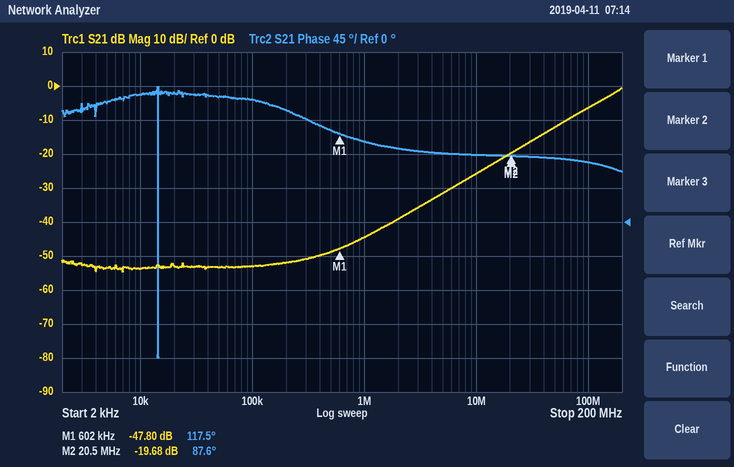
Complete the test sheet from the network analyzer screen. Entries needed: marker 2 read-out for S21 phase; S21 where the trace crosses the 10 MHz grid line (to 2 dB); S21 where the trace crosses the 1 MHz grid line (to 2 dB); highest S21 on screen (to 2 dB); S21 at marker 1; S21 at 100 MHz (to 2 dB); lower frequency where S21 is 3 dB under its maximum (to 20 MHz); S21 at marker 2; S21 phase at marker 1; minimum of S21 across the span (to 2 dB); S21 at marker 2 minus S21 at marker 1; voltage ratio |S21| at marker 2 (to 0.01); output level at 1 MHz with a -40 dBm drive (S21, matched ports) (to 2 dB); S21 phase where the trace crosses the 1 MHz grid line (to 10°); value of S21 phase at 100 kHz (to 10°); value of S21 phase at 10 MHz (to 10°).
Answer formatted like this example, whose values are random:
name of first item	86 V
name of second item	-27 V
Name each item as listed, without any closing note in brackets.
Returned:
marker 2 read-out for S21 phase	87.6°
S21 where the trace crosses the 10 MHz grid line	-26 dB
S21 where the trace crosses the 1 MHz grid line	-44 dB
highest S21 on screen	0 dB
S21 at marker 1	-47.80 dB
S21 at 100 MHz	-6 dB
lower frequency where S21 is 3 dB under its maximum	140 MHz
S21 at marker 2	-19.68 dB
S21 phase at marker 1	117.5°
minimum of S21 across the span	-54 dB
S21 at marker 2 minus S21 at marker 1	28.12 dB
voltage ratio |S21| at marker 2	0.10
output level at 1 MHz with a -40 dBm drive (S21, matched ports)	-84 dBm
S21 phase where the trace crosses the 1 MHz grid line	110°
value of S21 phase at 100 kHz	160°
value of S21 phase at 10 MHz	90°
